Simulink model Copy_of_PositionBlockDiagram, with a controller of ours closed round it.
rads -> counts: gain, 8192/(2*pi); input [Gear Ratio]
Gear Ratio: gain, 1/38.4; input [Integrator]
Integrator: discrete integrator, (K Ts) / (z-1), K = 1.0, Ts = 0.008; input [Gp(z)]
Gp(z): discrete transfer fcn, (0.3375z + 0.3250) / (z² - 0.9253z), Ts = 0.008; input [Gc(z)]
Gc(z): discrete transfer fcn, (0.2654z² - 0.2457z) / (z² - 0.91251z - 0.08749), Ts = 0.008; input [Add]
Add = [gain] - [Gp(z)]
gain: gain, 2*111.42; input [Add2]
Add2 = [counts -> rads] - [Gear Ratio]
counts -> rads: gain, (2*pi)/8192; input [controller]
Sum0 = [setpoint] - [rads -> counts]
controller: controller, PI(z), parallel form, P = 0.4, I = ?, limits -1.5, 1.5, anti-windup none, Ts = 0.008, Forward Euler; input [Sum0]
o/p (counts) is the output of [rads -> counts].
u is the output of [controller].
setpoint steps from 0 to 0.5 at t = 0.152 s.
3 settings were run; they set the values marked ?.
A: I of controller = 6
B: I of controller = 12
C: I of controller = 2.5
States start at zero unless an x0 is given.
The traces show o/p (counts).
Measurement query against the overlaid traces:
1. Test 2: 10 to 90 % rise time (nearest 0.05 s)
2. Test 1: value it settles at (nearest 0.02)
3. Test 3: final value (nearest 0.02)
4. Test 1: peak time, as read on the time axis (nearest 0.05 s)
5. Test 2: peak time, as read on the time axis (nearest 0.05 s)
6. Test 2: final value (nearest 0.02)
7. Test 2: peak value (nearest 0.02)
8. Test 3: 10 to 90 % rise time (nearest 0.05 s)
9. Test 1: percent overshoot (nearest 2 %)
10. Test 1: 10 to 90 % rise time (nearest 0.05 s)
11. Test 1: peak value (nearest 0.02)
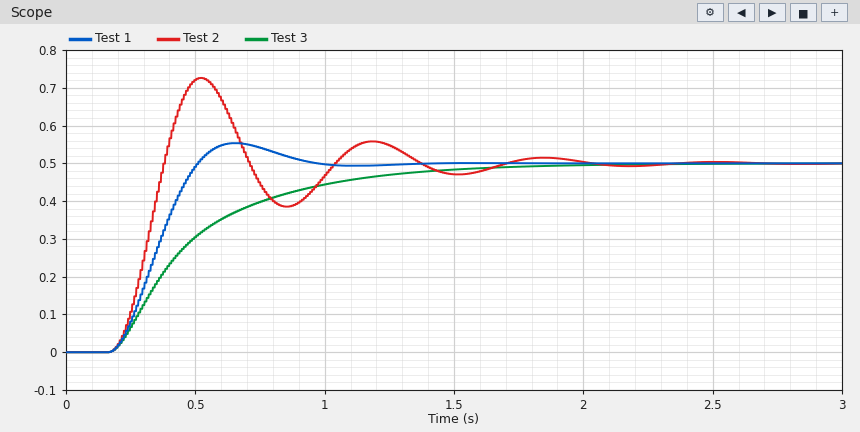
0.15 s
0.50
0.50
0.65 s
0.50 s
0.50
0.72
0.80 s
10 %
0.25 s
0.56
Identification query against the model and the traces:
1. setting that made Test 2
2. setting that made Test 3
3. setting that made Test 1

B
C
A
